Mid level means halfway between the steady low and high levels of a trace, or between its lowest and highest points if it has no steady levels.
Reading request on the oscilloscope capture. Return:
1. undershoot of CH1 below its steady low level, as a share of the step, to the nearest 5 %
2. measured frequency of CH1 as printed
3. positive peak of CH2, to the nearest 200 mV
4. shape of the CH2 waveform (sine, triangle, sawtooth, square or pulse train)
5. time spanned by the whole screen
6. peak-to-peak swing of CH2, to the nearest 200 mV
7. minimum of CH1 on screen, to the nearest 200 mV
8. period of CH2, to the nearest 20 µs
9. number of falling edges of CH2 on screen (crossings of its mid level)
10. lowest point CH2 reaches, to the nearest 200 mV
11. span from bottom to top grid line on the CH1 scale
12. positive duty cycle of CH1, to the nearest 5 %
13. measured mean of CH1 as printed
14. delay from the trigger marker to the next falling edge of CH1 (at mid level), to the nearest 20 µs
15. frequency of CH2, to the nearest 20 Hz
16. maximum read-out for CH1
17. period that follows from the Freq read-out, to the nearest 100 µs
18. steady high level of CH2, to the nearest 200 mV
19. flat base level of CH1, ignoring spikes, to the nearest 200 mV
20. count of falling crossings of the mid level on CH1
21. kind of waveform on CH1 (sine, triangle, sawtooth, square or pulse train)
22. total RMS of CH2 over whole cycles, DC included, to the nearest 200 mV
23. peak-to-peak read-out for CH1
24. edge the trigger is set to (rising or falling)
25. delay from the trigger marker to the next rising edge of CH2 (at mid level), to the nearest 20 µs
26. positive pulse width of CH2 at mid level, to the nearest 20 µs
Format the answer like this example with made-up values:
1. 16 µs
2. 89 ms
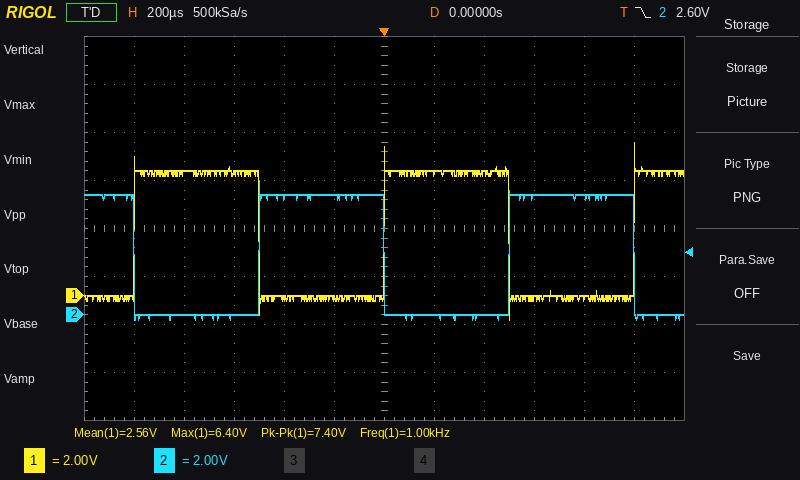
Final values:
1. 20 %
2. 1.00 kHz
3. 5.6 V
4. square
5. 2.4 ms
6. 5.8 V
7. -1.0 V
8. 1.00 ms
9. 3
10. -200 mV
11. 16 V
12. 50 %
13. 2.56 V
14. 500 µs
15. 1.00 kHz
16. 6.40 V
17. 1.0 ms
18. 5.0 V
19. 0.0 V
20. 2
21. square
22. 3.6 V
23. 7.40 V
24. falling
25. 500 µs
26. 500 µs
